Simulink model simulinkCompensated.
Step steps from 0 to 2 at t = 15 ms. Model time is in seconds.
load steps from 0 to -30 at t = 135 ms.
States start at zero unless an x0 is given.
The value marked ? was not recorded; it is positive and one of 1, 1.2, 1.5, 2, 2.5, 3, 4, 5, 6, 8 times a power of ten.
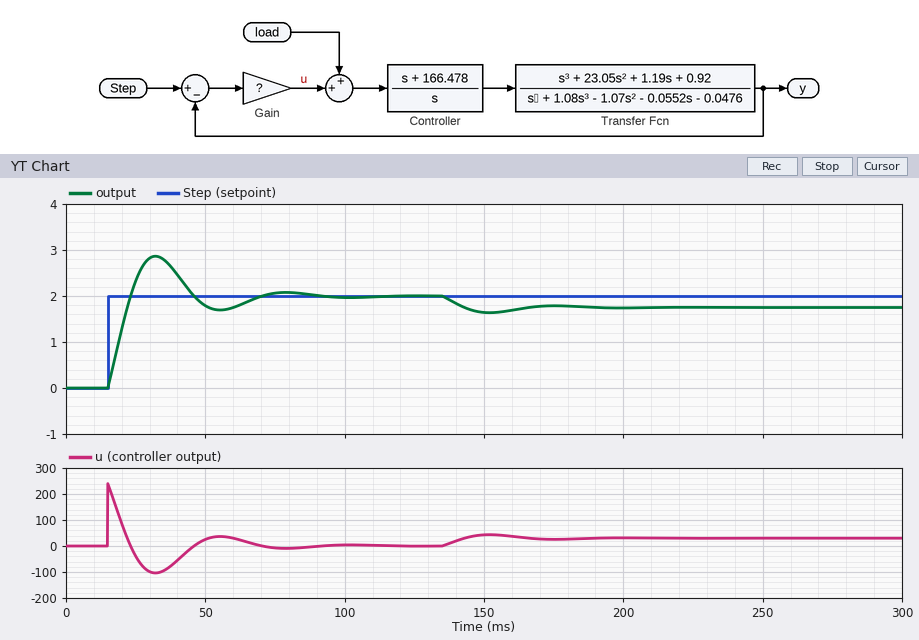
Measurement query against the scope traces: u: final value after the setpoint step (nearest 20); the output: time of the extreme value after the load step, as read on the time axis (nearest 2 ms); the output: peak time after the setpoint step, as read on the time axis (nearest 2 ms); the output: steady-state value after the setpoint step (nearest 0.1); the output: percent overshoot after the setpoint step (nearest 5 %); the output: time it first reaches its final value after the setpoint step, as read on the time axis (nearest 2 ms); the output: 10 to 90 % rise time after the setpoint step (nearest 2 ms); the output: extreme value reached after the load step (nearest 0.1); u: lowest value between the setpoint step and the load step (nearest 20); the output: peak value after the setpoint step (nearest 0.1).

0
152 ms
32 ms
2.0
45 %
24 ms
6 ms
1.6
-100
2.9
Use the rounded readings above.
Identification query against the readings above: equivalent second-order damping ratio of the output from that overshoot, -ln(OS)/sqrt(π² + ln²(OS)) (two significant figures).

0.25
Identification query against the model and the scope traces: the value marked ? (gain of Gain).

120
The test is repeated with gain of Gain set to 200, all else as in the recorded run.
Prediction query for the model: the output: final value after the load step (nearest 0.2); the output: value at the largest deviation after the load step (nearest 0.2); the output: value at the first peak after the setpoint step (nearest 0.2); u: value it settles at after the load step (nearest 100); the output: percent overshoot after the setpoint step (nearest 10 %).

1.8
1.8
2.6
0
30 %
